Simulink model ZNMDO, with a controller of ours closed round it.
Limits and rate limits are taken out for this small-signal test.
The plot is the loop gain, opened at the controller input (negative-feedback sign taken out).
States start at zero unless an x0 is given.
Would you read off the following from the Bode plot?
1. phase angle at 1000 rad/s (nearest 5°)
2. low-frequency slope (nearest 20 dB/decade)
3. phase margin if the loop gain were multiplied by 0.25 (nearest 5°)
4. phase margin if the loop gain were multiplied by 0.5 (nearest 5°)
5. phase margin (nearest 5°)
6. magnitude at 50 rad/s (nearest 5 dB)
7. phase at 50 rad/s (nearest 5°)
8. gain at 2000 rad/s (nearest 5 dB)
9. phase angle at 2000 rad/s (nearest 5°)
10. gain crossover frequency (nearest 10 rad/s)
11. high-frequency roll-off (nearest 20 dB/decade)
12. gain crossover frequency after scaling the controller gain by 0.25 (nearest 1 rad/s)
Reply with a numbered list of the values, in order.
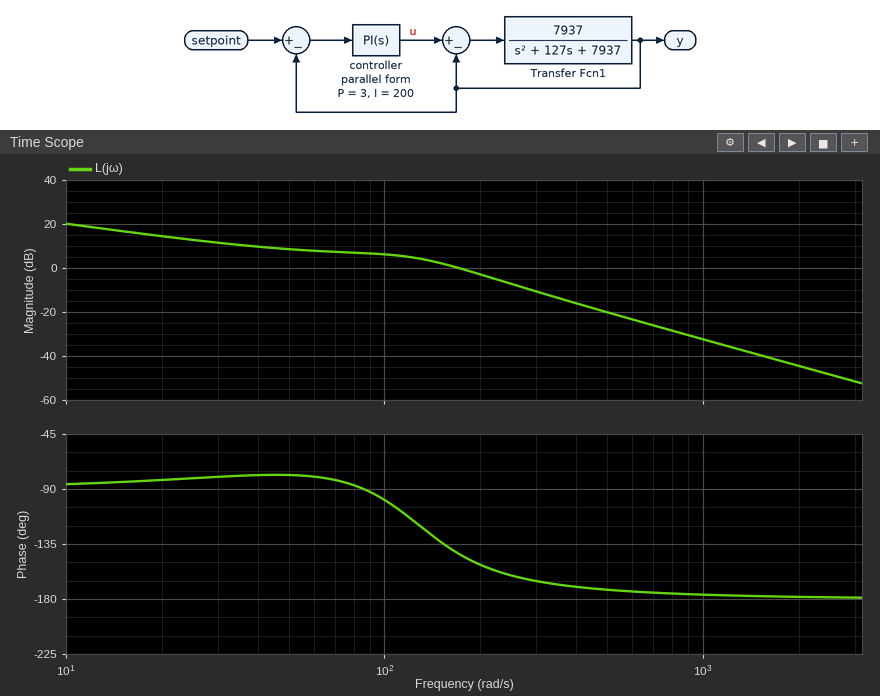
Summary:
1. -175°
2. -20 dB/decade
3. 100°
4. 80°
5. 35°
6. 10 dB
7. -80°
8. -45 dB
9. -180°
10. 170 rad/s
11. -40 dB/decade
12. 28 rad/s
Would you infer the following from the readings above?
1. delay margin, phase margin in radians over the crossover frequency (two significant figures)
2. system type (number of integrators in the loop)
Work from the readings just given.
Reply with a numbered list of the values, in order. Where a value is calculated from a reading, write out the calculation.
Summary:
1. 35 × π / 180 / 170 = 0.0036 s
2. 1
